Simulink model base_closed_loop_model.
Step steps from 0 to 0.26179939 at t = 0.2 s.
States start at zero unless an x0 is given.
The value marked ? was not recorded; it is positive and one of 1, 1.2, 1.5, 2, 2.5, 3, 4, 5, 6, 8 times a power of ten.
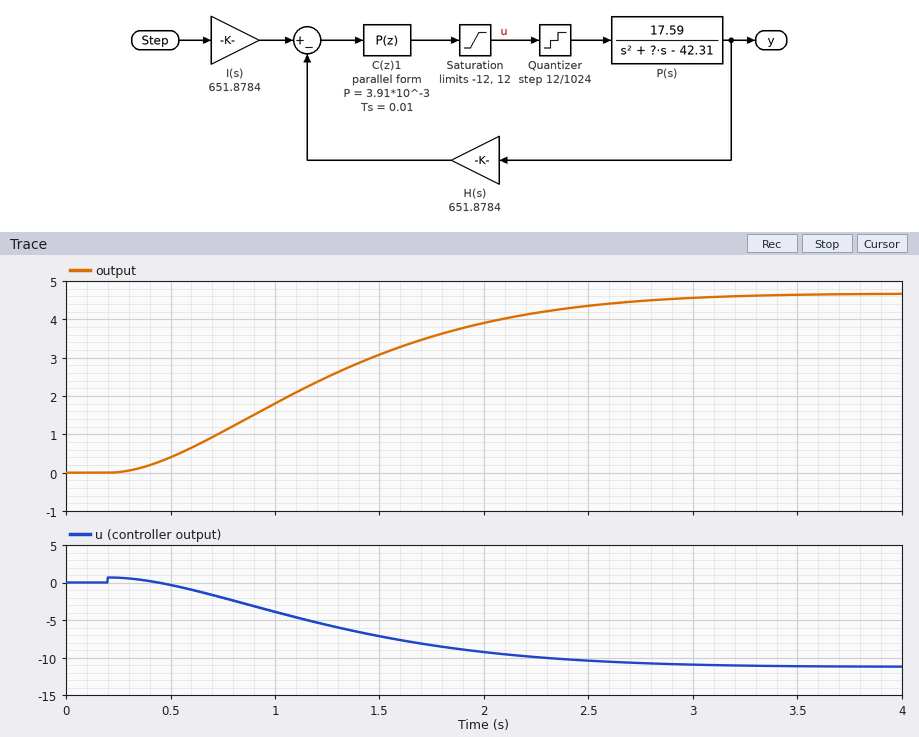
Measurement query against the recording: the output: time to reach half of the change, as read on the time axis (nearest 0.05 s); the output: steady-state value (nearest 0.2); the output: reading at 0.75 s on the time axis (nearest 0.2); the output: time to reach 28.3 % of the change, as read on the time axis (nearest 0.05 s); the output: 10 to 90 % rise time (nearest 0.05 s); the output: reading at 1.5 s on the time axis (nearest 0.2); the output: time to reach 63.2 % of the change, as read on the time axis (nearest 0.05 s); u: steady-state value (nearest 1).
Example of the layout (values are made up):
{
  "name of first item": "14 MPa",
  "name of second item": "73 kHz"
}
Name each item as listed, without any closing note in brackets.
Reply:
{
  "the output: time to reach half of the change, as read on the time axis": "1.20 s",
  "the output: steady-state value": "4.6",
  "the output: reading at 0.75 s on the time axis": "1.0",
  "the output: time to reach 28.3 % of the change, as read on the time axis": "0.85 s",
  "the output: 10 to 90 % rise time": "1.75 s",
  "the output: reading at 1.5 s on the time axis": "3.0",
  "the output: time to reach 63.2 % of the change, as read on the time axis": "1.45 s",
  "u: steady-state value": "-11"
}
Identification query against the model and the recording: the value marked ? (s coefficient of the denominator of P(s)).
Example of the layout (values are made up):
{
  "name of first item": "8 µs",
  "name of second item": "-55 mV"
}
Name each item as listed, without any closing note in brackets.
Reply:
{
  "the value marked ? (s coefficient of the denominator of P(s))": "3"
}
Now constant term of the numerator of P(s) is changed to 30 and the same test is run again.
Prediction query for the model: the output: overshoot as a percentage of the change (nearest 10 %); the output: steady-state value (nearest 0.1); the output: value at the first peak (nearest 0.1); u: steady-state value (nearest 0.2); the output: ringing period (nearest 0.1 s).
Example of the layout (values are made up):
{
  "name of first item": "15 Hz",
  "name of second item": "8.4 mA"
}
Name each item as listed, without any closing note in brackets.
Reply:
{
  "the output: overshoot as a percentage of the change": "50 %",
  "the output: steady-state value": "0.6",
  "the output: value at the first peak": "0.9",
  "u: steady-state value": "-0.8",
  "the output: ringing period": "1.1 s"
}
